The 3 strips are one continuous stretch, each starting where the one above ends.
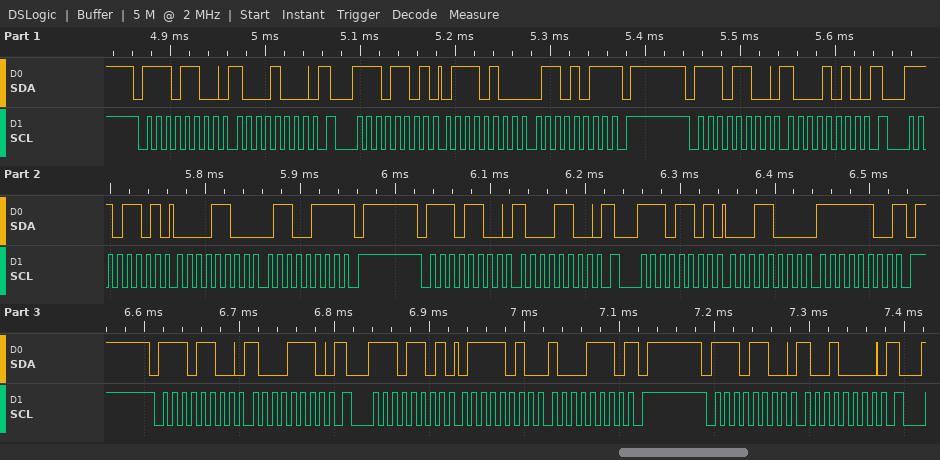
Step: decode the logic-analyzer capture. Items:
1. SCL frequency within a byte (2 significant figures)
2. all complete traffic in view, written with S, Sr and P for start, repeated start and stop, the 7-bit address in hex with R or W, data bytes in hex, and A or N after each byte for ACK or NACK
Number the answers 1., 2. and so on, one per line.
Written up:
1. 100 kHz
2. S 76W A 88 A Sr 76R A 74 A 6B N P S 76W A 8A A Sr 76R A 0C A 67 N P S 76W A 8C A Sr 76R A 18 A FC N P S 76W A 8E A Sr 76R A 7A A 8E N P S 76W A 90 A
